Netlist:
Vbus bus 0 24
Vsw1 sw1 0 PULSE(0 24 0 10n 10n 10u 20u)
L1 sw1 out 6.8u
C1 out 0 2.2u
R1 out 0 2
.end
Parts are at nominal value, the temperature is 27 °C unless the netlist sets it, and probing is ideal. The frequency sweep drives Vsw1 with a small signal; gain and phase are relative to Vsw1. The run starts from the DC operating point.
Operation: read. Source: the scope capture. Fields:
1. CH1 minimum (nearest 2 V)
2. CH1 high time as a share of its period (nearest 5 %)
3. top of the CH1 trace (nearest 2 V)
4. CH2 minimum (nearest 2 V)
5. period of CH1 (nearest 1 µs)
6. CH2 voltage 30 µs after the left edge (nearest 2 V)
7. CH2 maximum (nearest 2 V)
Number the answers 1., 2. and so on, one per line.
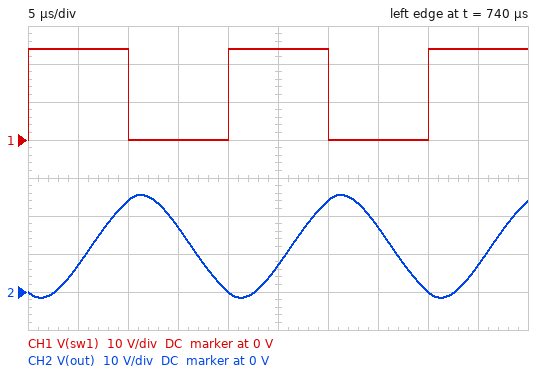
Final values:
1. 0 V
2. 50 %
3. 24 V
4. -2 V
5. 20 µs
6. 24 V
7. 26 V
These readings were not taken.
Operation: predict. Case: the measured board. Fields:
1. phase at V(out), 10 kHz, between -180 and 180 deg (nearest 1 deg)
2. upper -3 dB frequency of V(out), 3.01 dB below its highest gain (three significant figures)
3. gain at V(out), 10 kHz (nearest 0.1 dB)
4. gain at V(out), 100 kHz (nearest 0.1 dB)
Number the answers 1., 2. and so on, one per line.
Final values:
1. -13 deg
2. 48.7 kHz
3. 0.3 dB
4. -14.6 dB
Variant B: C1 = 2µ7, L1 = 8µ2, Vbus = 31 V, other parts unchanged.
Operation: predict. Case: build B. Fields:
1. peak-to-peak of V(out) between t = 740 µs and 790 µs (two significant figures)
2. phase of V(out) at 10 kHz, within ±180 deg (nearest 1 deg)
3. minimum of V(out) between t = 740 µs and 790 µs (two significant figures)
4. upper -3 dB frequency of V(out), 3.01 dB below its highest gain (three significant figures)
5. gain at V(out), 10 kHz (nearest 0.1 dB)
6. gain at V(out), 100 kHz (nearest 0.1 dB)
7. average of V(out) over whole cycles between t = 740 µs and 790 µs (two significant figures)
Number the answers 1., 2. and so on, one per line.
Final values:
1. 18 V
2. -16 deg
3. 3.1 V
4. 40.1 kHz
5. 0.5 dB
6. -18.2 dB
7. 12 V
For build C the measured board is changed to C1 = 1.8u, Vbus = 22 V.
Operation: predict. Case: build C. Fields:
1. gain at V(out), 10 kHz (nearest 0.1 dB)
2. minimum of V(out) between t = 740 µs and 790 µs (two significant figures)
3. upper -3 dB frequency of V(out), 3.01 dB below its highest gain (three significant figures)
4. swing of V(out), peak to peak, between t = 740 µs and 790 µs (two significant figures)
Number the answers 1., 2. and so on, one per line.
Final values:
1. 0.2 dB
2. -2.6 V
3. 53.4 kHz
4. 29 V
